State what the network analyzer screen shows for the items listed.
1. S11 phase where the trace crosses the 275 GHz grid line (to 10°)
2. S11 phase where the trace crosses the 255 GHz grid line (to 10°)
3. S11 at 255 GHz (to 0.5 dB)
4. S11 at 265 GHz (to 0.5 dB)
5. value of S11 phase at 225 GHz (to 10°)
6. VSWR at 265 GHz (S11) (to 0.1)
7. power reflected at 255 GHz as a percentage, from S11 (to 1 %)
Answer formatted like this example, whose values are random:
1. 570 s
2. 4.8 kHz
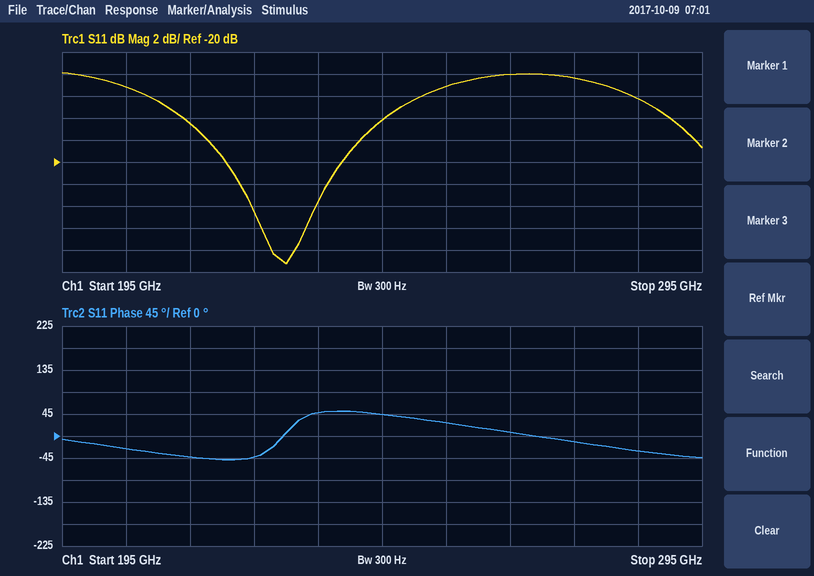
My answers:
1. -10°
2. 30°
3. -13.0 dB
4. -12.0 dB
5. -40°
6. 1.7
7. 5 %
